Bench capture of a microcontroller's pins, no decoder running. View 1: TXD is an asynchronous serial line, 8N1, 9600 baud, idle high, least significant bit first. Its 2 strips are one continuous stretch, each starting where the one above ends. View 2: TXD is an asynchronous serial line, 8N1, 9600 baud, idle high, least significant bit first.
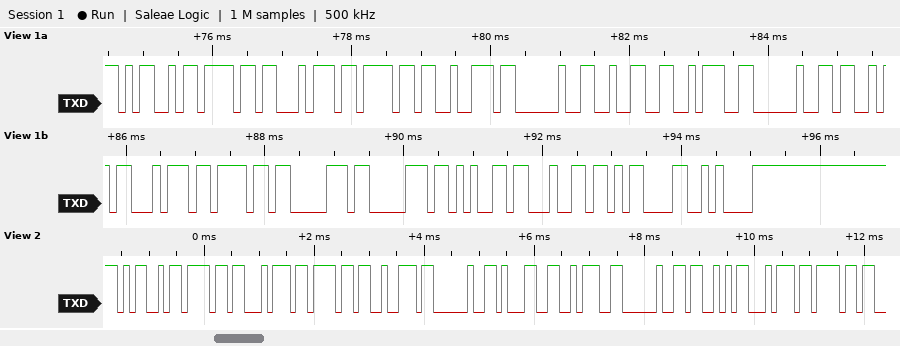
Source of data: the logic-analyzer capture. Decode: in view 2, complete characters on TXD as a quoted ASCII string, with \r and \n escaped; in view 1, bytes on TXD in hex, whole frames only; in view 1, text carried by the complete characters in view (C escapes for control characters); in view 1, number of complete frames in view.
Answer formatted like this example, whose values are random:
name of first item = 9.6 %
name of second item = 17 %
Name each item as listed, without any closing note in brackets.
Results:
in view 2, complete characters on TXD as a quoted ASCII string, with \r and \n escaped = "Motor 1: Sto"
in view 1, bytes on TXD in hex, whole frames only = 0x4D 0x6F 0x74 0x6F 0x72 0x20 0x32 0x3A 0x20 0x53 0x74 0x6F 0x70 0x70 0x65 0x64 0x0D 0x0A
in view 1, text carried by the complete characters in view = "Motor 2: Stopped\r\n"
in view 1, number of complete frames in view = 18
